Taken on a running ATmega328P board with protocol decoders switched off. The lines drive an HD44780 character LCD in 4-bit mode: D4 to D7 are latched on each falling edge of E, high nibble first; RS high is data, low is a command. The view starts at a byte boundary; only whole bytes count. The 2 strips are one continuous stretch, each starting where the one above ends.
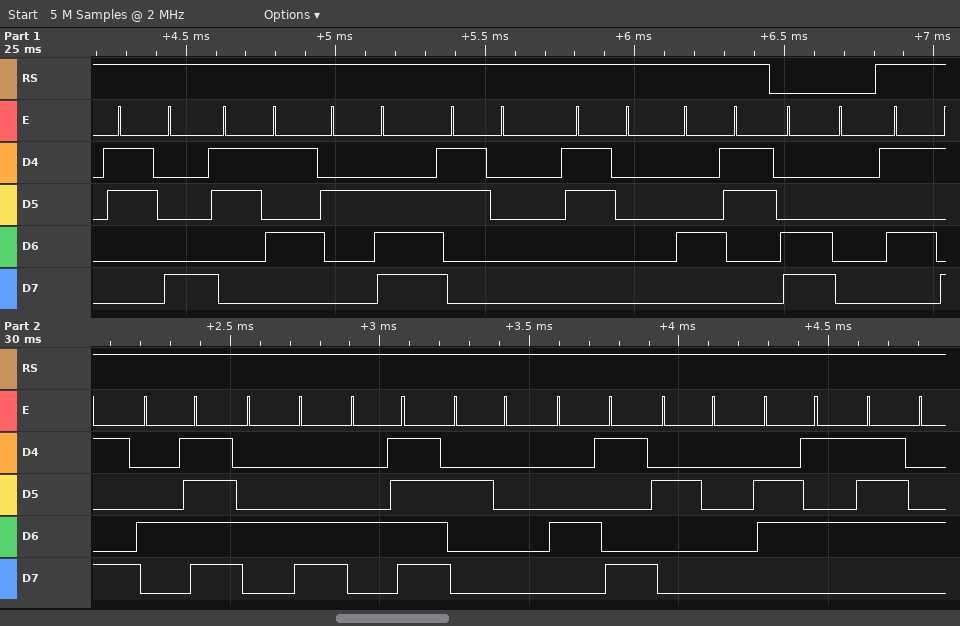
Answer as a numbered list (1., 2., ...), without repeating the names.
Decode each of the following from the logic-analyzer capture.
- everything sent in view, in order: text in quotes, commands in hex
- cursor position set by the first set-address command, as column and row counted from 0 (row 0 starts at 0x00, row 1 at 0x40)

1. "85.00C" 0xC0 "YOLO I et"
2. column 0, row 1
